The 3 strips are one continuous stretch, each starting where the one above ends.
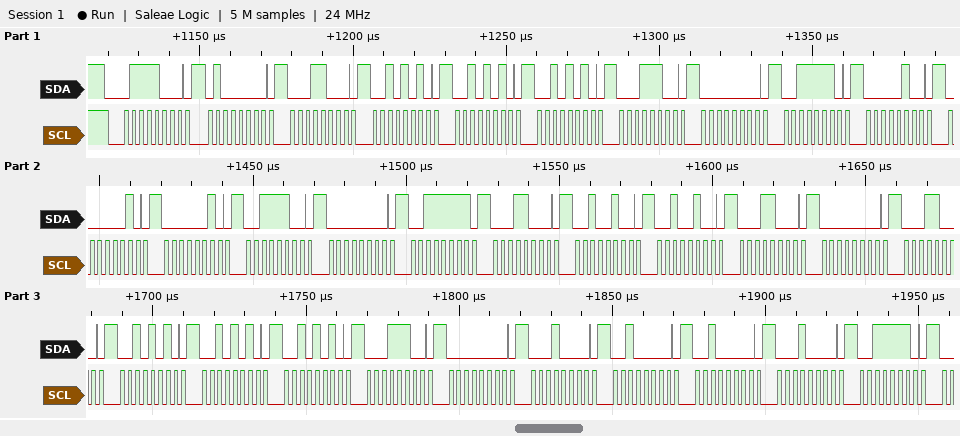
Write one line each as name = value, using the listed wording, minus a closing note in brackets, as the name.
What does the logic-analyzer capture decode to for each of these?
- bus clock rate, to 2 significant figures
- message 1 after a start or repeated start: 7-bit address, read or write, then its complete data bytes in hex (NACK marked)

bus clock rate, to 2 significant figures = 400 kHz
message 1 after a start or repeated start: 7-bit address, read or write, then its complete data bytes in hex = 0x3C write: 40 18 2A 2A 2A 1C 00 3E 04 02 02 3C 00 3F 18 24 24 18 00 18 2A 2A 2A 1C 00 10 20 20 10 3E
